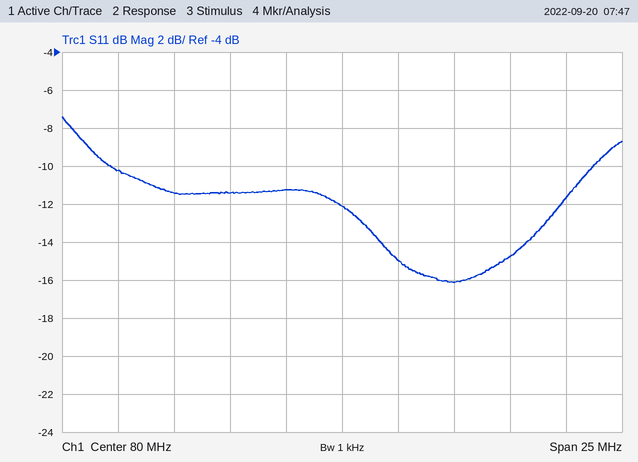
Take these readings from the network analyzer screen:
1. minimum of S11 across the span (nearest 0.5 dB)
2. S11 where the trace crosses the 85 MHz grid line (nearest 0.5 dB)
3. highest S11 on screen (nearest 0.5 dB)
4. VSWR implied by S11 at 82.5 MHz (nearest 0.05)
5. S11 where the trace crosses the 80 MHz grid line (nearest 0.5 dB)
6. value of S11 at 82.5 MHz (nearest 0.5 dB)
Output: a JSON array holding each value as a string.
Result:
["-16.0 dB", "-16.0 dB", "-7.5 dB", "1.45", "-12.0 dB", "-15.0 dB"]
